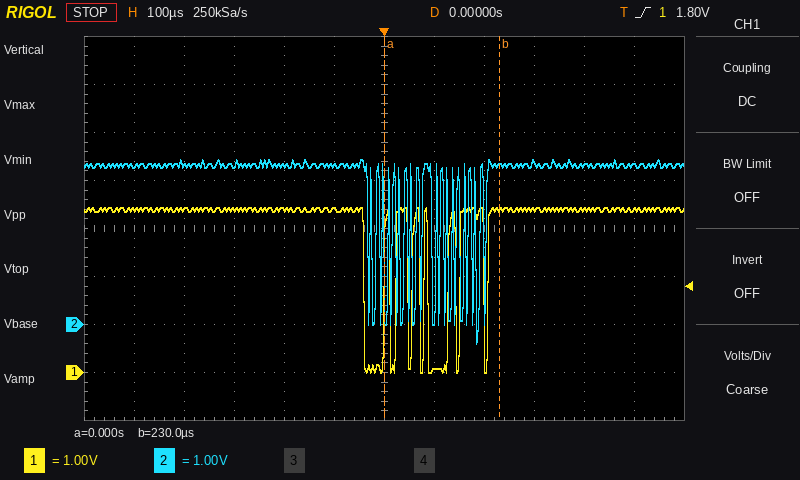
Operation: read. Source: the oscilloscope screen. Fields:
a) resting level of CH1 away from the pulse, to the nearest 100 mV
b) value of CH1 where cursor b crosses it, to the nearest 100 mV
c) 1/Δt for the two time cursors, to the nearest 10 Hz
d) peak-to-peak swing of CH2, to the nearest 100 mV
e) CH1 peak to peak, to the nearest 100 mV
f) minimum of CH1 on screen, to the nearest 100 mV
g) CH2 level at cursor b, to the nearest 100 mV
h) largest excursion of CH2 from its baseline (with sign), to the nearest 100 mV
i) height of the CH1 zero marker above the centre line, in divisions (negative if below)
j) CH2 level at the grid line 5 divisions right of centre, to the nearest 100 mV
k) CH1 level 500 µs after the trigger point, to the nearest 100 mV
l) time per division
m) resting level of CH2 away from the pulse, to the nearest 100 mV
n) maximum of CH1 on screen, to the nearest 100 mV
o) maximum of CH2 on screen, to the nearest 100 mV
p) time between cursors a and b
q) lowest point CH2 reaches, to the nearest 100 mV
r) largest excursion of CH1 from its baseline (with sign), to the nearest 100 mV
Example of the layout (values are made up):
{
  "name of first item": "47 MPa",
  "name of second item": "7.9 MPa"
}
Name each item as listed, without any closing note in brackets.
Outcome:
{
  "resting level of CH1 away from the pulse, to the nearest 100 mV": "3.4 V",
  "value of CH1 where cursor b crosses it, to the nearest 100 mV": "3.4 V",
  "1/Δt for the two time cursors, to the nearest 10 Hz": "4.35 kHz",
  "peak-to-peak swing of CH2, to the nearest 100 mV": "3.8 V",
  "CH1 peak to peak, to the nearest 100 mV": "3.4 V",
  "minimum of CH1 on screen, to the nearest 100 mV": "0.0 V",
  "CH2 level at cursor b, to the nearest 100 mV": "3.3 V",
  "largest excursion of CH2 from its baseline (with sign), to the nearest 100 mV": "-3.7 V",
  "height of the CH1 zero marker above the centre line, in divisions": "-3.0 div",
  "CH2 level at the grid line 5 divisions right of centre, to the nearest 100 mV": "3.3 V",
  "CH1 level 500 µs after the trigger point, to the nearest 100 mV": "3.4 V",
  "time per division": "100 µs",
  "resting level of CH2 away from the pulse, to the nearest 100 mV": "3.3 V",
  "maximum of CH1 on screen, to the nearest 100 mV": "3.4 V",
  "maximum of CH2 on screen, to the nearest 100 mV": "3.4 V",
  "time between cursors a and b": "230 µs",
  "lowest point CH2 reaches, to the nearest 100 mV": "-400 mV",
  "largest excursion of CH1 from its baseline (with sign), to the nearest 100 mV": "-3.4 V"
}
